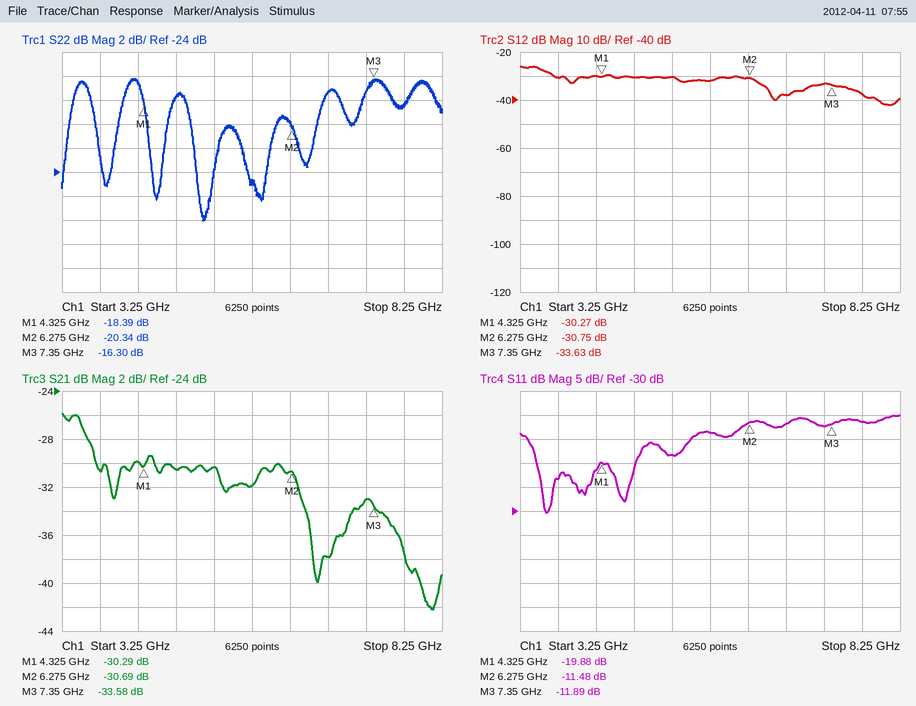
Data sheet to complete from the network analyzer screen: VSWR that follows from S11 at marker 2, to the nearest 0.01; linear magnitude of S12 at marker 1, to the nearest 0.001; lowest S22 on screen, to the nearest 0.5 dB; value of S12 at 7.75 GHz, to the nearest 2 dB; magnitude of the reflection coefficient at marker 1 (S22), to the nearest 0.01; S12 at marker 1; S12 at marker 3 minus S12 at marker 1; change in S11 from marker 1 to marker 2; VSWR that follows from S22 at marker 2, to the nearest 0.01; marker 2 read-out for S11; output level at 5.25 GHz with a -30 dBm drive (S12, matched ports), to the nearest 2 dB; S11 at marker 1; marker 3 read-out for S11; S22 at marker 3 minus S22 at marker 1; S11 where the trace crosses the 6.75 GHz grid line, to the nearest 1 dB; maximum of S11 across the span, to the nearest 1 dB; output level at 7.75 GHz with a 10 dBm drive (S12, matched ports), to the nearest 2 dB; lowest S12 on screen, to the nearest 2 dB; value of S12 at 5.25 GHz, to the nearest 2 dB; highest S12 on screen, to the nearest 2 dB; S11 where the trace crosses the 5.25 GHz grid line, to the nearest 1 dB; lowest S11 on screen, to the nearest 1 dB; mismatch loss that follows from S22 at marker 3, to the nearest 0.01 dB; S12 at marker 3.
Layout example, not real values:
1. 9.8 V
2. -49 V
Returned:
1. 1.73
2. 0.031
3. -28.0 dB
4. -38 dB
5. 0.12
6. -30.27 dB
7. -3.36 dB
8. 8.40 dB
9. 1.21
10. -11.48 dB
11. -60 dBm
12. -19.88 dB
13. -11.89 dB
14. 2.09 dB
15. -12 dB
16. -10 dB
17. -28 dBm
18. -42 dB
19. -30 dB
20. -26 dB
21. -18 dB
22. -30 dB
23. 0.10 dB
24. -33.63 dB
